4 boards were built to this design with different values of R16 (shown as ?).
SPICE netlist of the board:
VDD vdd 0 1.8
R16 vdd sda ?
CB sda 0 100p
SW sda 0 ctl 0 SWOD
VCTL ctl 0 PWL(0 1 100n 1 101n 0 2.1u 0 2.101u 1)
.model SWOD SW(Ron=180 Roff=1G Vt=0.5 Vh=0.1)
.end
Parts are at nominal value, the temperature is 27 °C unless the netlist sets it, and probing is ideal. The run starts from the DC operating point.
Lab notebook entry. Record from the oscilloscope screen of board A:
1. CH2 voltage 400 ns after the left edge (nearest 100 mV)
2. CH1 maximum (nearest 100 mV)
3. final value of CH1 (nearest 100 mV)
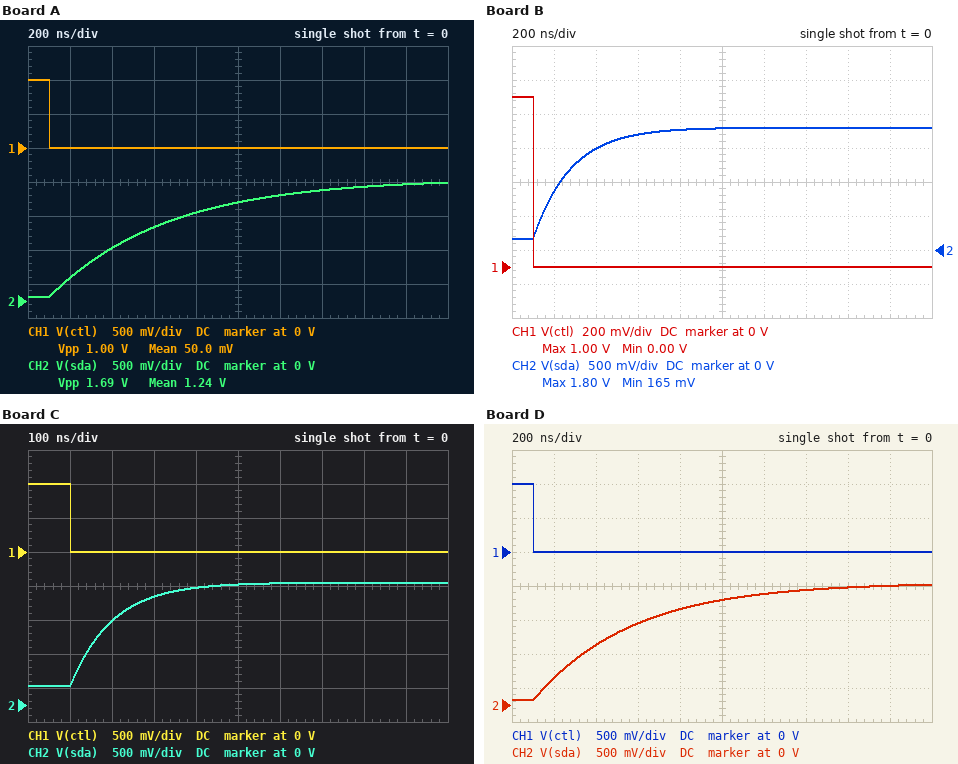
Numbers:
800 mV
1.0 V
0 V
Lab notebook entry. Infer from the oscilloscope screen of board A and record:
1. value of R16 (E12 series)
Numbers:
5.6 kΩ
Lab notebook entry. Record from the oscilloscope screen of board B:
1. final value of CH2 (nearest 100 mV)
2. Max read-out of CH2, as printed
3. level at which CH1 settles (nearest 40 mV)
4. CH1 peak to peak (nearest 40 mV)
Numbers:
1.8 V
1.80 V
0 V
1.00 V
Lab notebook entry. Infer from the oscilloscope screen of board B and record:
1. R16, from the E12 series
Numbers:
1.8 kΩ
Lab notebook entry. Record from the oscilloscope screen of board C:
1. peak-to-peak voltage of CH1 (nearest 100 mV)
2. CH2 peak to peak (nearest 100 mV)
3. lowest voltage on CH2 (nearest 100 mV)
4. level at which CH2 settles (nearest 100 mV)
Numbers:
1.0 V
1.5 V
300 mV
1.8 V
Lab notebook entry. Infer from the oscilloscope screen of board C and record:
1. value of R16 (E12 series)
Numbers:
1 kΩ
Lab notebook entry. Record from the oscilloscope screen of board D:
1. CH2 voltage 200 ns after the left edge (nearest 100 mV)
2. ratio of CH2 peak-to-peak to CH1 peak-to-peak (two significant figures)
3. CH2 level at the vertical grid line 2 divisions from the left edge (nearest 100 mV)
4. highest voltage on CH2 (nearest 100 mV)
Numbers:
400 mV
1.7
900 mV
1.8 V
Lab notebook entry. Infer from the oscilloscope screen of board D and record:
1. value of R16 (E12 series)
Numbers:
4.7 kΩ
